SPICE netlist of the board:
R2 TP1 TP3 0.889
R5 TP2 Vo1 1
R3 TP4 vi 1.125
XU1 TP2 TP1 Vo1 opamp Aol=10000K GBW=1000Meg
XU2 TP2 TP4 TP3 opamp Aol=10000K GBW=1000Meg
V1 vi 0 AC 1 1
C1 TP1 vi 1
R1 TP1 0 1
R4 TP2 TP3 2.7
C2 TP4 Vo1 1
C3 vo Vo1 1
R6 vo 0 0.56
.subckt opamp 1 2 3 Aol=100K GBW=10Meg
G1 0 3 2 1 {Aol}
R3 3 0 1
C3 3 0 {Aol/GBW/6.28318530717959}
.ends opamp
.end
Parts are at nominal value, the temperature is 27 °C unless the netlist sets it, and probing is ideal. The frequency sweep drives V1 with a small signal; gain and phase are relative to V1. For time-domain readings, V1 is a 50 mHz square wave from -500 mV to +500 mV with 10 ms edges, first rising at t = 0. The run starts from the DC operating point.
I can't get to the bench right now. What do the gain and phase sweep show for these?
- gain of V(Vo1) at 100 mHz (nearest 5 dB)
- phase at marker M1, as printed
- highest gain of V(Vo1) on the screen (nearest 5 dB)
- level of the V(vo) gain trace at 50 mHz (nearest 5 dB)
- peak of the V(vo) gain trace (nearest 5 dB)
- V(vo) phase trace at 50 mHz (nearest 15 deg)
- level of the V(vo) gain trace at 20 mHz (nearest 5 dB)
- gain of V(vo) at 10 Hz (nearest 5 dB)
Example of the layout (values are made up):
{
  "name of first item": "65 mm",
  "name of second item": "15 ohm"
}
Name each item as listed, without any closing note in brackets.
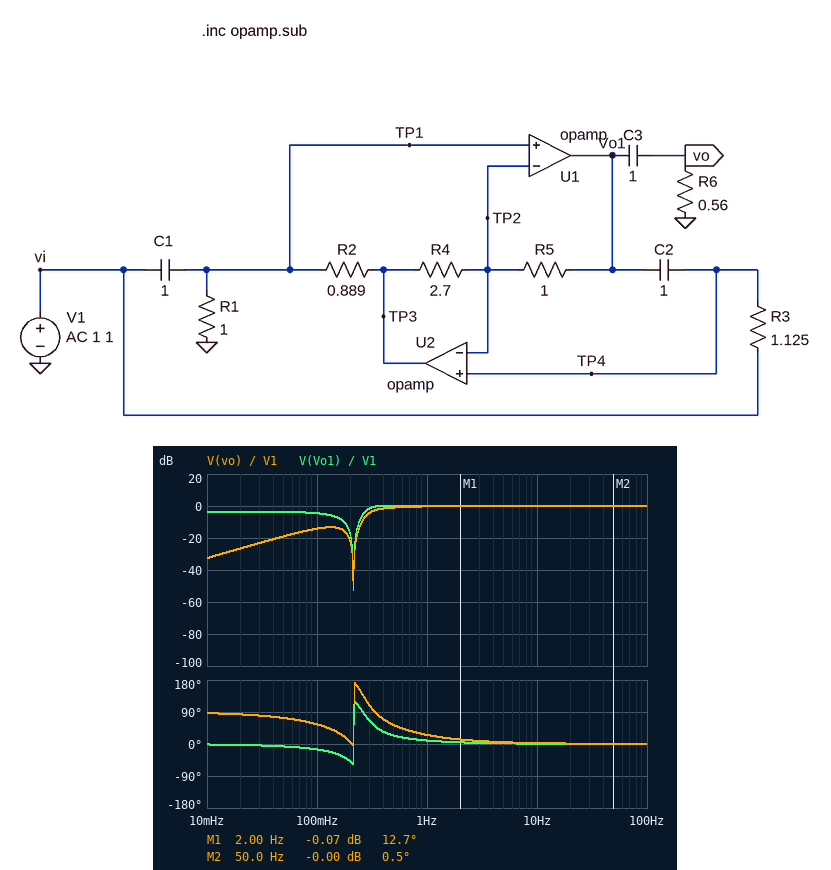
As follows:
{
  "gain of V(Vo1) at 100 mHz": "-5 dB",
  "phase at marker M1, as printed": "12.7 deg",
  "highest gain of V(Vo1) on the screen": "0 dB",
  "level of the V(vo) gain trace at 50 mHz": "-20 dB",
  "peak of the V(vo) gain trace": "0 dB",
  "V(vo) phase trace at 50 mHz": "75 deg",
  "level of the V(vo) gain trace at 20 mHz": "-25 dB",
  "gain of V(vo) at 10 Hz": "0 dB"
}
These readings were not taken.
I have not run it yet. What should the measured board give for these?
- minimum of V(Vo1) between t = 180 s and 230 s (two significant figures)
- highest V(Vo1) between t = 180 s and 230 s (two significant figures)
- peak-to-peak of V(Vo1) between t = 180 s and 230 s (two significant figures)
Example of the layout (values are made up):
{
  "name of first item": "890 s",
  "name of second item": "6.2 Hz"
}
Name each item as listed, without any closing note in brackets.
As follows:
{
  "minimum of V(Vo1) between t = 180 s and 230 s": "-660 mV",
  "highest V(Vo1) between t = 180 s and 230 s": "660 mV",
  "peak-to-peak of V(Vo1) between t = 180 s and 230 s": "1.3 V"
}
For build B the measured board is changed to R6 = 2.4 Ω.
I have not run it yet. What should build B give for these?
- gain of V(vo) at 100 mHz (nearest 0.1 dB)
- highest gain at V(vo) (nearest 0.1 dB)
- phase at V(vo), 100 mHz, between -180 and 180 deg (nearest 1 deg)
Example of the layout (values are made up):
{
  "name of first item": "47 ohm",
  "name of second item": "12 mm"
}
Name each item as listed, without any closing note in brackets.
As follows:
{
  "gain of V(vo) at 100 mHz": "-6.1 dB",
  "highest gain at V(vo)": "0.2 dB",
  "phase at V(vo), 100 mHz, between -180 and 180 deg": "18 deg"
}
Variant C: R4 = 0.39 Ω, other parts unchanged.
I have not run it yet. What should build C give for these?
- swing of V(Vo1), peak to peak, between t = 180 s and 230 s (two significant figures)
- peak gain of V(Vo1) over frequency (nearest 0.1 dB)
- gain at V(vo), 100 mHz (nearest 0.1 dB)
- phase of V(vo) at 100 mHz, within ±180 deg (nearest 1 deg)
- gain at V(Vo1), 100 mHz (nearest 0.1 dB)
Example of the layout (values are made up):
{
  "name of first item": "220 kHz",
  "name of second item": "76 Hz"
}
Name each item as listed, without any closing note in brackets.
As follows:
{
  "swing of V(Vo1), peak to peak, between t = 180 s and 230 s": "3.3 V",
  "peak gain of V(Vo1) over frequency": "3.2 dB",
  "gain at V(vo), 100 mHz": "-6.5 dB",
  "phase of V(vo) at 100 mHz, within ±180 deg": "160 deg",
  "gain at V(Vo1), 100 mHz": "3.1 dB"
}
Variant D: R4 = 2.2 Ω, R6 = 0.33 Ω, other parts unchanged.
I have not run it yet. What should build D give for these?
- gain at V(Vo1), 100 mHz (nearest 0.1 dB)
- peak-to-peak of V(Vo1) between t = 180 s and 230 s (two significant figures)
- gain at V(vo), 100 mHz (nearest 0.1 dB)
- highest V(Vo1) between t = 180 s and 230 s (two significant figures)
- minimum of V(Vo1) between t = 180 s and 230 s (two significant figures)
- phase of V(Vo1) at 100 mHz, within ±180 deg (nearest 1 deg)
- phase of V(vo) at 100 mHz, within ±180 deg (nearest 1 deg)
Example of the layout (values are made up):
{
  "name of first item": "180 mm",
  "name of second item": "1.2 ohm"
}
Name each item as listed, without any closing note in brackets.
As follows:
{
  "gain at V(Vo1), 100 mHz": "-6.4 dB",
  "peak-to-peak of V(Vo1) between t = 180 s and 230 s": "1.4 V",
  "gain at V(vo), 100 mHz": "-20.2 dB",
  "highest V(Vo1) between t = 180 s and 230 s": "700 mV",
  "minimum of V(Vo1) between t = 180 s and 230 s": "-700 mV",
  "phase of V(Vo1) at 100 mHz, within ±180 deg": "-19 deg",
  "phase of V(vo) at 100 mHz, within ±180 deg": "59 deg"
}
